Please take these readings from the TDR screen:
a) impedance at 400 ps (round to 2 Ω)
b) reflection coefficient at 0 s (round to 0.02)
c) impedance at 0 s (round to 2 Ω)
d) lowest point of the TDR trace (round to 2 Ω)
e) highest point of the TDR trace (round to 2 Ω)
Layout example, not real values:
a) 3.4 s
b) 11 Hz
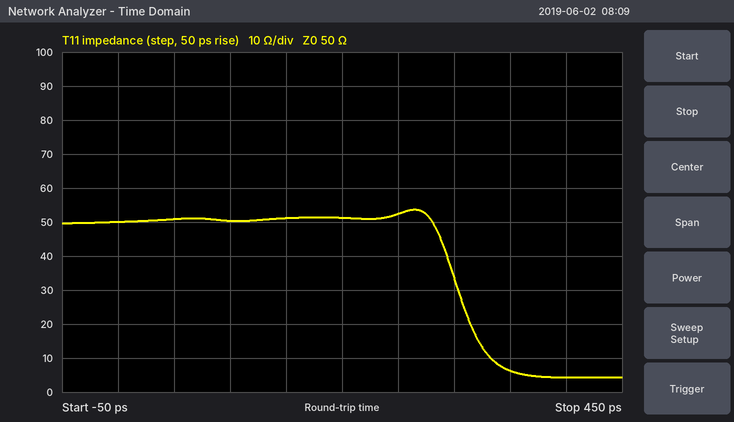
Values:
a) 4 Ω
b) 0.00
c) 50 Ω
d) 4 Ω
e) 54 Ω
